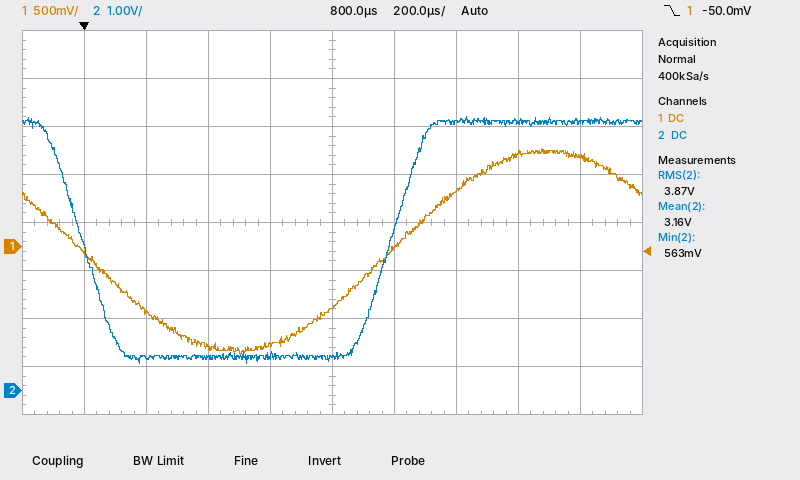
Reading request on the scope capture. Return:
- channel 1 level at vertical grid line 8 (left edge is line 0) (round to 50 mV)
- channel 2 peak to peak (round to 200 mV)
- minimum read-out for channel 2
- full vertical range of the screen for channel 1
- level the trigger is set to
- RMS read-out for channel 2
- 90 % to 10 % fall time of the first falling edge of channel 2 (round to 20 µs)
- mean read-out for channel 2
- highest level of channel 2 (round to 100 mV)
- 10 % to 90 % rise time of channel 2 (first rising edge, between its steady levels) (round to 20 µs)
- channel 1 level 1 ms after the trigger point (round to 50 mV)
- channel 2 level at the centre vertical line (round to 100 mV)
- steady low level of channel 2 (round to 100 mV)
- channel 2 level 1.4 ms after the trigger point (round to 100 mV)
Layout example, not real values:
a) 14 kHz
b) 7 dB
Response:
a) 950 mV
b) 5.2 V
c) 563 mV
d) 4 V
e) -50.0 mV
f) 3.87 V
g) 200 µs
h) 3.16 V
i) 5.7 V
j) 200 µs
k) 0 mV
l) 700 mV
m) 700 mV
n) 5.6 V
